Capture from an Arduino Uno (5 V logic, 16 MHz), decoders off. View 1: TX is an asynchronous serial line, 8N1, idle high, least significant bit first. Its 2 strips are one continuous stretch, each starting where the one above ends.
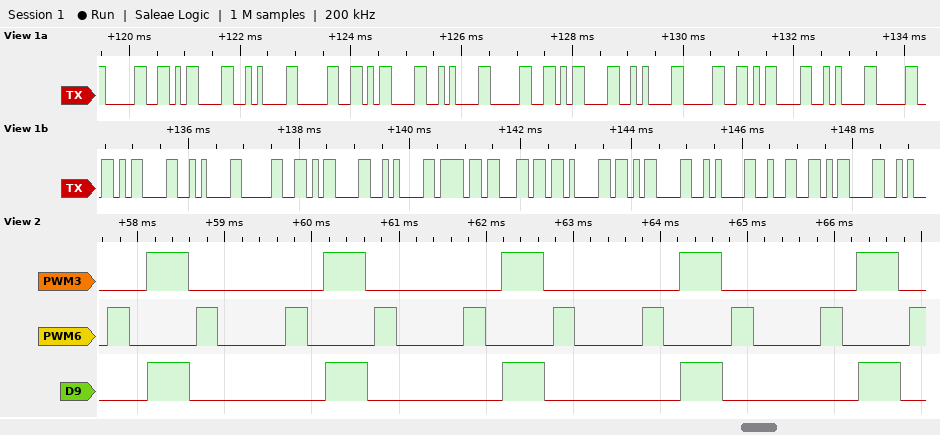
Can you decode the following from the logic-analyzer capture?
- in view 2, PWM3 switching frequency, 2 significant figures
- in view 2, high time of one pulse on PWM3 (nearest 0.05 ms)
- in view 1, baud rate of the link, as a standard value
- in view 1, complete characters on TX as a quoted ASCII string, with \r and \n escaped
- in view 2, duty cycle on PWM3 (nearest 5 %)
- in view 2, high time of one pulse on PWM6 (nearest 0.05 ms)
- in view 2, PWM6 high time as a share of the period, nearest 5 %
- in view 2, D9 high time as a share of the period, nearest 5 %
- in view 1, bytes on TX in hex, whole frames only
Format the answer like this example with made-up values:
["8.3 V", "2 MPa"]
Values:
["490 Hz", "0.50 ms", "9600 baud", "\"0\\r\\n0\\r\\n0\\r\\n0\\r\\n0\\r\\n0\\r\\nola\\r\\n2\\r\"", "25 %", "0.25 ms", "25 %", "25 %", "30 0D 0A 30 0D 0A 30 0D 0A 30 0D 0A 30 0D 0A 30 0D 0A 6F 6C 61 0D 0A 32 0D"]
